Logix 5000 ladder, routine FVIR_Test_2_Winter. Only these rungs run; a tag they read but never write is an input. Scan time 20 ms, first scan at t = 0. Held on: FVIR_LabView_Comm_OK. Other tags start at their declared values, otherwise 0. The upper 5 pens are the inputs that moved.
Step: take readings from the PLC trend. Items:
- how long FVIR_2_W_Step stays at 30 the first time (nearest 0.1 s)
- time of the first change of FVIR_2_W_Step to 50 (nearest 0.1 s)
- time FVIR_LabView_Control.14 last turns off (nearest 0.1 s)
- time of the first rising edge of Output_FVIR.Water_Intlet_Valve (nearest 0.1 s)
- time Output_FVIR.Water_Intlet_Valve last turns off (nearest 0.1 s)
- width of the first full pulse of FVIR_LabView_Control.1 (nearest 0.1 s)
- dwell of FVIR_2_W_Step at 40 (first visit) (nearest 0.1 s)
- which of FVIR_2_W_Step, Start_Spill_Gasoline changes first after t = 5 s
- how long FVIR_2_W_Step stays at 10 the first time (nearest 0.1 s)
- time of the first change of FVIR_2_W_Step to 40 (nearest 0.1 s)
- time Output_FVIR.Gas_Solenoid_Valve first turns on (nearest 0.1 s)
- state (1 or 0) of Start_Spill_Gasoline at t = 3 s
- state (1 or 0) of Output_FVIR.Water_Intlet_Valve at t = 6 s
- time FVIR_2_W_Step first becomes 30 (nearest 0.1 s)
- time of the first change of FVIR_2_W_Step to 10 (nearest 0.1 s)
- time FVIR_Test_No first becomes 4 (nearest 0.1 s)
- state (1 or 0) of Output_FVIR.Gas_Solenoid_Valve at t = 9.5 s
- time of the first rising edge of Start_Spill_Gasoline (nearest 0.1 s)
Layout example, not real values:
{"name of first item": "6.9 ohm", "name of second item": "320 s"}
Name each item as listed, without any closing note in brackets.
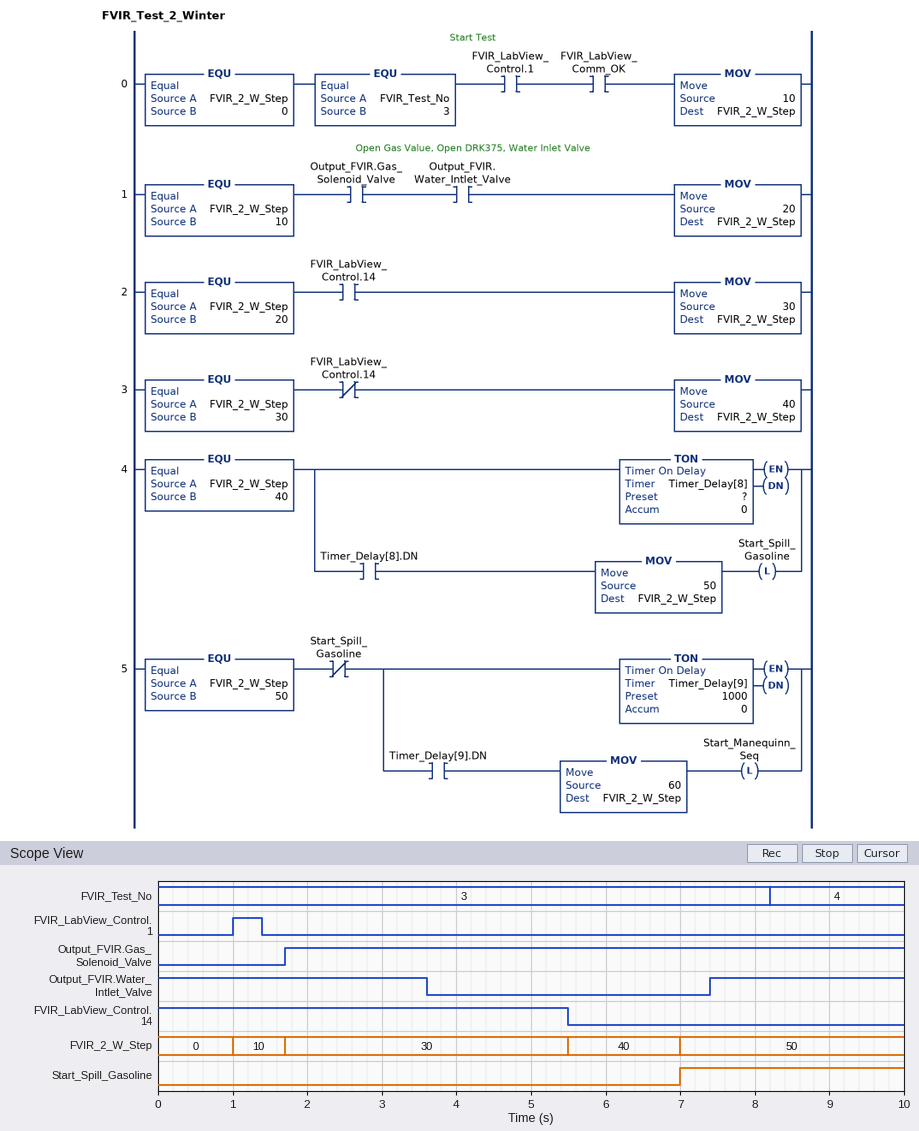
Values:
{"how long FVIR_2_W_Step stays at 30 the first time": "3.8 s", "time of the first change of FVIR_2_W_Step to 50": "7.0 s", "time FVIR_LabView_Control.14 last turns off": "5.5 s", "time of the first rising edge of Output_FVIR.Water_Intlet_Valve": "7.4 s", "time Output_FVIR.Water_Intlet_Valve last turns off": "3.6 s", "width of the first full pulse of FVIR_LabView_Control.1": "0.4 s", "dwell of FVIR_2_W_Step at 40 (first visit)": "1.5 s", "which of FVIR_2_W_Step, Start_Spill_Gasoline changes first after t = 5 s": "FVIR_2_W_Step", "how long FVIR_2_W_Step stays at 10 the first time": "0.7 s", "time of the first change of FVIR_2_W_Step to 40": "5.5 s", "time Output_FVIR.Gas_Solenoid_Valve first turns on": "1.7 s", "state (1 or 0) of Start_Spill_Gasoline at t = 3 s": "0", "state (1 or 0) of Output_FVIR.Water_Intlet_Valve at t = 6 s": "0", "time FVIR_2_W_Step first becomes 30": "1.7 s", "time of the first change of FVIR_2_W_Step to 10": "1.0 s", "time FVIR_Test_No first becomes 4": "8.2 s", "state (1 or 0) of Output_FVIR.Gas_Solenoid_Valve at t = 9.5 s": "1", "time of the first rising edge of Start_Spill_Gasoline": "7.0 s"}
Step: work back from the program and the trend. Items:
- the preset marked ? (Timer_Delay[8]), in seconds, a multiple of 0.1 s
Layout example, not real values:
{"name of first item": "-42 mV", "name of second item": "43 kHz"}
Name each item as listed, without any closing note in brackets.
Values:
{"the preset marked ? (Timer_Delay[8]), in seconds, a multiple of 0.1 s": "1.5 s"}
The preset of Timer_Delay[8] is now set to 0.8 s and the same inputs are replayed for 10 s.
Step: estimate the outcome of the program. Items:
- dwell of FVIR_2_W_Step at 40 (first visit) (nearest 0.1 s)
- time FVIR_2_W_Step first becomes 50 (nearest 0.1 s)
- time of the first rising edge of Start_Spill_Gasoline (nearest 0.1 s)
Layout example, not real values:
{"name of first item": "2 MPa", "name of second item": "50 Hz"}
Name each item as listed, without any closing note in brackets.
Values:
{"dwell of FVIR_2_W_Step at 40 (first visit)": "0.8 s", "time FVIR_2_W_Step first becomes 50": "6.3 s", "time of the first rising edge of Start_Spill_Gasoline": "6.3 s"}
